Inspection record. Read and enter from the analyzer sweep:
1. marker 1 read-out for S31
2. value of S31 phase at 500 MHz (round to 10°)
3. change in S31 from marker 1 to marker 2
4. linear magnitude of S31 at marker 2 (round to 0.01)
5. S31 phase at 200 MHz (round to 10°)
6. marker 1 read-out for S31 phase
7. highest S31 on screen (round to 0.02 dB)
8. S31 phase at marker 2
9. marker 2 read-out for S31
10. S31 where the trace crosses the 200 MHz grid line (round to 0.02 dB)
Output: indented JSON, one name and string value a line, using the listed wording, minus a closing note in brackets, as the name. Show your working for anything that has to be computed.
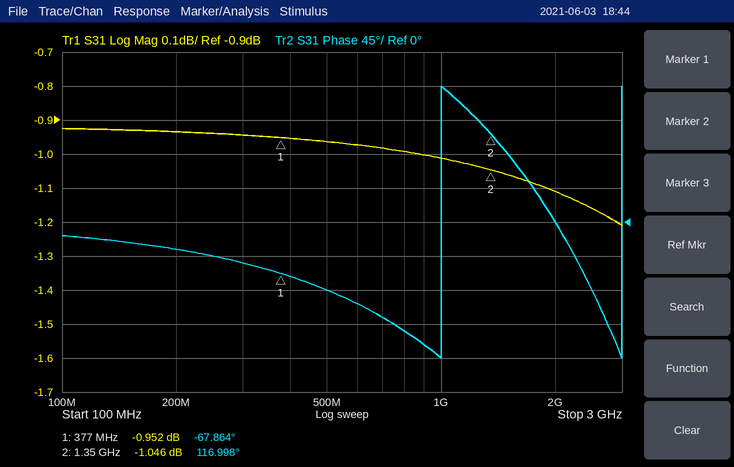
{
  "marker 1 read-out for S31": "-0.952 dB",
  "value of S31 phase at 500 MHz": "-90°",
  "change in S31 from marker 1 to marker 2": "-1.046 − (-0.952) = -0.094 dB",
  "linear magnitude of S31 at marker 2": "10^(-1.046/20) ≈ 0.89",
  "S31 phase at 200 MHz": "-40°",
  "marker 1 read-out for S31 phase": "-67.864°",
  "highest S31 on screen": "-0.92 dB",
  "S31 phase at marker 2": "116.998°",
  "marker 2 read-out for S31": "-1.046 dB",
  "S31 where the trace crosses the 200 MHz grid line": "-0.94 dB"
}
